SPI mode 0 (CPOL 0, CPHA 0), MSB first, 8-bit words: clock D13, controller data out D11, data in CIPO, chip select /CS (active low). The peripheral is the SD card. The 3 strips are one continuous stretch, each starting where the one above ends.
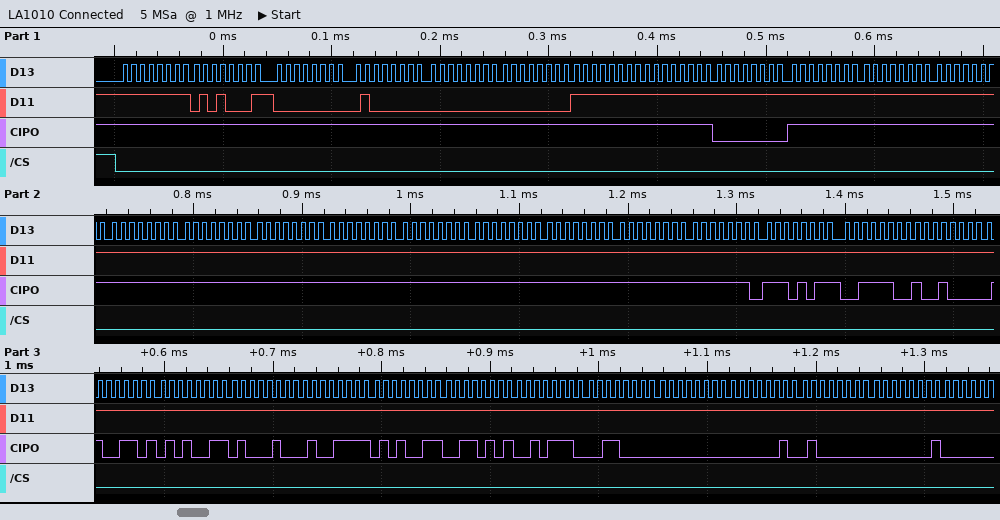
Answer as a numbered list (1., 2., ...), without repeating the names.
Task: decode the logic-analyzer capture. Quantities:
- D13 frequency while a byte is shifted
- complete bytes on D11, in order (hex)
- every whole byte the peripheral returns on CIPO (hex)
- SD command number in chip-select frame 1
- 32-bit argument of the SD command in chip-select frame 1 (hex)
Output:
1. 125 kHz
2. FF 51 00 40 00 00 FF FF FF FF FF FF FF FF FF FF FF FF FF FF FF FF FF FF FF FF FF FF FF FF FF FF FF FF FF FF
3. FF FF FF FF FF FF FF FF 00 FF FF FF FF FF FF FF FF FF FF FF FE EB 3C 90 4D 53 44 4F 53 35 2E 30 00 02 40 01
4. CMD17
5. 0x00400000
